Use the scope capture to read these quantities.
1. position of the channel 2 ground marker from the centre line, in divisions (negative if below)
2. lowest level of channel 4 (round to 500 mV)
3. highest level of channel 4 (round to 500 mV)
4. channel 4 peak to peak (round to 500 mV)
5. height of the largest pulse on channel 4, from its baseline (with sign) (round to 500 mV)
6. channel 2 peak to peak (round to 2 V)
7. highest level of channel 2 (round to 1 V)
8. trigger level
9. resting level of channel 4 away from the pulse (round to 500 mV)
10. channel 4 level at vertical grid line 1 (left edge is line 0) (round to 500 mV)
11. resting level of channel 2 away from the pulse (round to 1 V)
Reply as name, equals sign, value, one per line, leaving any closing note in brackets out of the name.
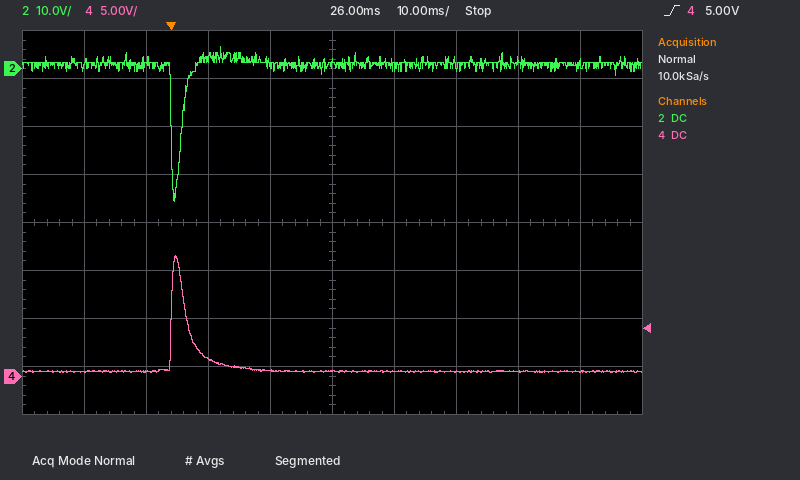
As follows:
position of the channel 2 ground marker from the centre line, in divisions = +3.2 div
lowest level of channel 4 = 500 mV
highest level of channel 4 = 12.5 V
channel 4 peak to peak = 12.0 V
height of the largest pulse on channel 4, from its baseline (with sign) = +12.0 V
channel 2 peak to peak = 32 V
highest level of channel 2 = 5 V
trigger level = 5.00 V
resting level of channel 4 away from the pulse = 500 mV
channel 4 level at vertical grid line 1 (left edge is line 0) = 500 mV
resting level of channel 2 away from the pulse = 1 V
